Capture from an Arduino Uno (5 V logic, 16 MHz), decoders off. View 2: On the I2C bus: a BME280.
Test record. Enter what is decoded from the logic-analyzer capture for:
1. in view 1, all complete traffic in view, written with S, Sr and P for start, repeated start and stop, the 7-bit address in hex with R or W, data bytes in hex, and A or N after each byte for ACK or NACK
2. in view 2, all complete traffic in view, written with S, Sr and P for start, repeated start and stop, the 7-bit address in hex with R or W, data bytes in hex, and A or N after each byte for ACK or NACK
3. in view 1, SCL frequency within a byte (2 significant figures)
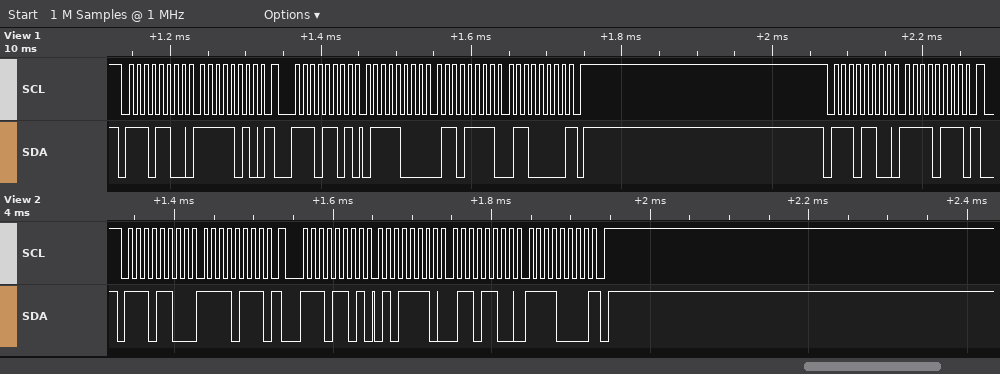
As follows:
S 76W A FA A Sr 76R A 78 A 6F A 60 N P S 76W A F7 A
S 76W A F7 A Sr 76R A 5E A 6C A F0 N P
100 kHz
